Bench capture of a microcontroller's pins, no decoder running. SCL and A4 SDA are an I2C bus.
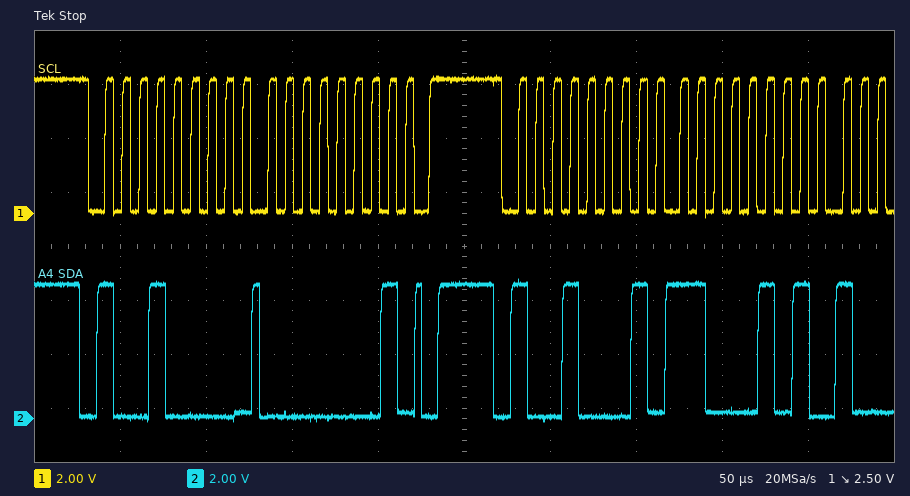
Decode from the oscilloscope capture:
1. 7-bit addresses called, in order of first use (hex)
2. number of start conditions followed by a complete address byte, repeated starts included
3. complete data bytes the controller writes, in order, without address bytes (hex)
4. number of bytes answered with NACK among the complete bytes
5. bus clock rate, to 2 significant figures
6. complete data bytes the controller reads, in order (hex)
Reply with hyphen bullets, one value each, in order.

- 0x48
- 2
- 01
- 0
- 100 kHz
- C5
